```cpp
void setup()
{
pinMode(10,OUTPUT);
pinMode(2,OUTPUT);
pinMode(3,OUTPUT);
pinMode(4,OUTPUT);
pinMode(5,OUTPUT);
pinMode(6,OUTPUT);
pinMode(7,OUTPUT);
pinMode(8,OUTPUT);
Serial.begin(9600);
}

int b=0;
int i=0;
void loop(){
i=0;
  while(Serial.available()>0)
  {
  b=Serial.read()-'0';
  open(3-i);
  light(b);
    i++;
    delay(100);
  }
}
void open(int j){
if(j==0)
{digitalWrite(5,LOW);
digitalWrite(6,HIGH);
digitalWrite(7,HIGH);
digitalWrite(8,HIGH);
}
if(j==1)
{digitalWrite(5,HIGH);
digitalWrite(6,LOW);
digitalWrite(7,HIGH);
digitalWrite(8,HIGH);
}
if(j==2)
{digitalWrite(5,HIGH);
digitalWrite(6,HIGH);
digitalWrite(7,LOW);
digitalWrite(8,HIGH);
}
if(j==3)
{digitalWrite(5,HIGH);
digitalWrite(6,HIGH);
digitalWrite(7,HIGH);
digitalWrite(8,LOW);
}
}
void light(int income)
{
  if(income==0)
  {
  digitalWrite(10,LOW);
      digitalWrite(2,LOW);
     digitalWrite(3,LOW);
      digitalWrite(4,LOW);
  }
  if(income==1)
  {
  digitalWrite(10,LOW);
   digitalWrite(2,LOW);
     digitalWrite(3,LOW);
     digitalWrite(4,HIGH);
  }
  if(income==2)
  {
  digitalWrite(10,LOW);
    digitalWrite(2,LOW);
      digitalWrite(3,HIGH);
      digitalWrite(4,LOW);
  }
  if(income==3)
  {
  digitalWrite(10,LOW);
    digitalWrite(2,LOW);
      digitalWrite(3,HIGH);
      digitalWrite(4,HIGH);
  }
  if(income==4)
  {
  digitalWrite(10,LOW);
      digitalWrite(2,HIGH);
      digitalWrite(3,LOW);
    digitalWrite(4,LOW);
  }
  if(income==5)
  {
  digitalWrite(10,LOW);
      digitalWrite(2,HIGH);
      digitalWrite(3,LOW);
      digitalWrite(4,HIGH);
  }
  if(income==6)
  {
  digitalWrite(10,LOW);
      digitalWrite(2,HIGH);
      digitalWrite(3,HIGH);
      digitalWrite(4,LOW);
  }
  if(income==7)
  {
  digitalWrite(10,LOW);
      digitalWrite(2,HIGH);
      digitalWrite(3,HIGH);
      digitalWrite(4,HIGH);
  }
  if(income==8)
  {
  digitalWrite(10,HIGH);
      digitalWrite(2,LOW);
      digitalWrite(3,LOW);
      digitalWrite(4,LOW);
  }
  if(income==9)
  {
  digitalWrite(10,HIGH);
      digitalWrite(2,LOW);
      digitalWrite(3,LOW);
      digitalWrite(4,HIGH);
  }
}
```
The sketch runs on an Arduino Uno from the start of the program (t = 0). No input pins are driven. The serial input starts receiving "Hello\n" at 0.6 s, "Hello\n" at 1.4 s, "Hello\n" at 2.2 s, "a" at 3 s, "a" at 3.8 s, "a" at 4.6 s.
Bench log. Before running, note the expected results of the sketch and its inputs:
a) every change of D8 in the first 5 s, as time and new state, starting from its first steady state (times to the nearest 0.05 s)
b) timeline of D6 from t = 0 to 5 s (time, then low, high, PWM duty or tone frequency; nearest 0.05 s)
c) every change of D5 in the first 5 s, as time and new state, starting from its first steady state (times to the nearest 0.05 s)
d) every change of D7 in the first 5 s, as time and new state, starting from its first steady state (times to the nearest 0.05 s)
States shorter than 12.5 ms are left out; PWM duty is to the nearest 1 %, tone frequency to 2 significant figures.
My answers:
0 s low; 0.7 s high; 1.4 s low; 1.5 s high; 2.2 s low; 2.3 s high; 3 s low
0 s low; 0.6 s high; 0.8 s low; 0.9 s high; 1.6 s low; 1.7 s high; 2.4 s low; 2.5 s high
0 s low; 0.6 s high; 0.9 s low; 1.4 s high; 1.7 s low; 2.2 s high; 2.5 s low; 3 s high
0 s low; 0.6 s high; 0.7 s low; 0.8 s high; 1.5 s low; 1.6 s high; 2.3 s low; 2.4 s high
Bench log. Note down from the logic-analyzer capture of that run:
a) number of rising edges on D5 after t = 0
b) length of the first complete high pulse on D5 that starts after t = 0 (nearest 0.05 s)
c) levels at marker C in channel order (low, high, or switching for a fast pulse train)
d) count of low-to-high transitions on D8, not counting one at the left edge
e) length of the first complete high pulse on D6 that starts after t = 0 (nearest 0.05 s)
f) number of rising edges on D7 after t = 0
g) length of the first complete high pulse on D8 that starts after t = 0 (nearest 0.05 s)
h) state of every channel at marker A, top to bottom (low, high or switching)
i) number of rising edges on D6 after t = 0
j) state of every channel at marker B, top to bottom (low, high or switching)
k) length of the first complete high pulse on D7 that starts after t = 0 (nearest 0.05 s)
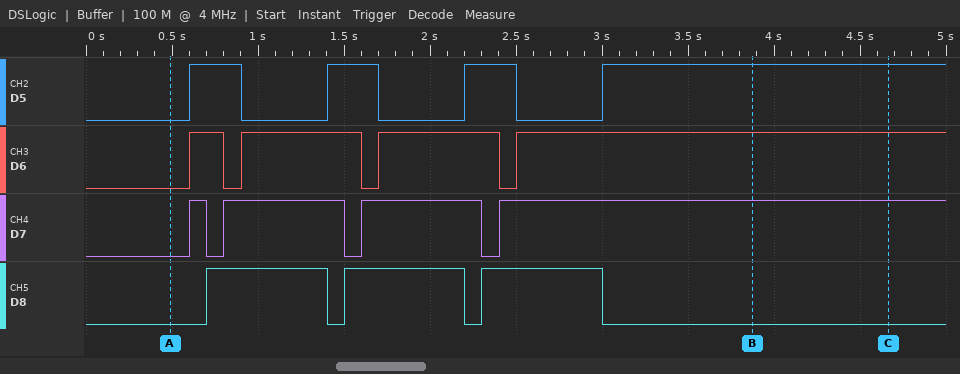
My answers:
4
0.30 s
D5 high, D6 high, D7 high, D8 low
3
0.20 s
4
0.70 s
D5 low, D6 low, D7 low, D8 low
4
D5 high, D6 high, D7 high, D8 low
0.10 s
